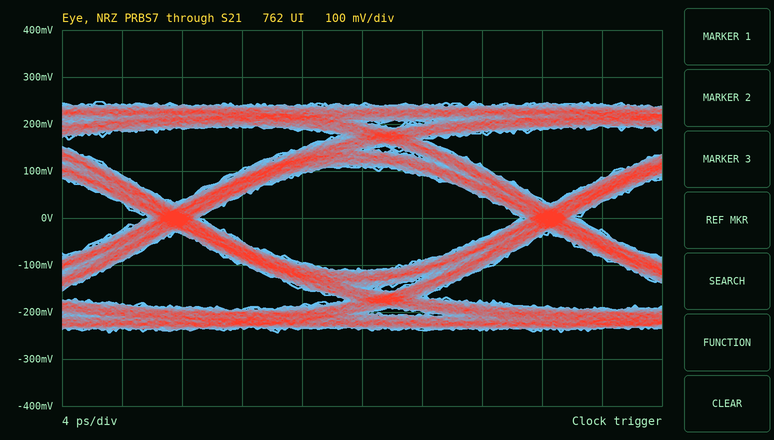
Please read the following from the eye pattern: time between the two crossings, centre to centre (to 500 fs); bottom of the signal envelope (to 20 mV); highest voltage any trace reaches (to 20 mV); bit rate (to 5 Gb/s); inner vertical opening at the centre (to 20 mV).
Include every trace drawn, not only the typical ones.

25.0 ps
-240 mV
240 mV
40 Gb/s
220 mV
